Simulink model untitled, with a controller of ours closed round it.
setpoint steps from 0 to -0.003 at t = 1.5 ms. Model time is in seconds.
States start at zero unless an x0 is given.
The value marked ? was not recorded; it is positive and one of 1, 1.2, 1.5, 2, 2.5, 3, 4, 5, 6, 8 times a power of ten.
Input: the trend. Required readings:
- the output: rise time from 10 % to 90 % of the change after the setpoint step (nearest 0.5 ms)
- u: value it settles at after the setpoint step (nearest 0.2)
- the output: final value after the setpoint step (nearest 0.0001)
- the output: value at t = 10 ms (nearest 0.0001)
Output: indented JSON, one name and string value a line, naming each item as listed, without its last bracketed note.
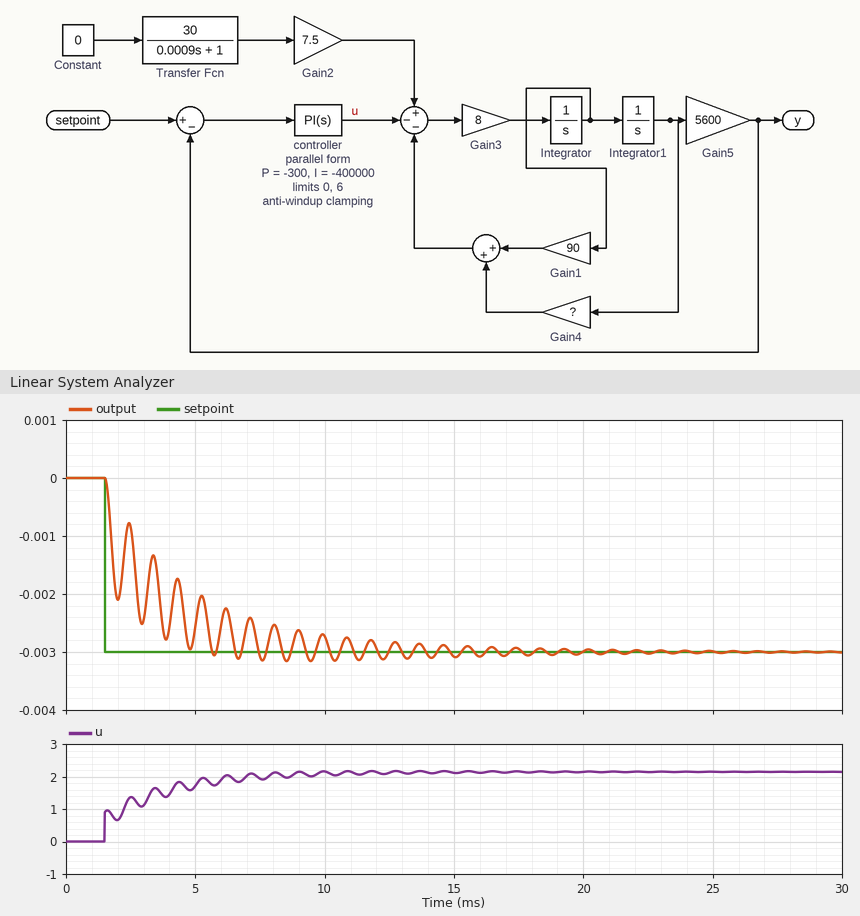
{
  "the output: rise time from 10 % to 90 % of the change after the setpoint step": "2.0 ms",
  "u: value it settles at after the setpoint step": "2.2",
  "the output: final value after the setpoint step": "-0.0030",
  "the output: value at t = 10 ms": "-0.0027"
}
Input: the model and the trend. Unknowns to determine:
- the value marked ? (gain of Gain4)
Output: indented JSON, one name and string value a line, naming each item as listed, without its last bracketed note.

{
  "the value marked ?": "4e+06"
}
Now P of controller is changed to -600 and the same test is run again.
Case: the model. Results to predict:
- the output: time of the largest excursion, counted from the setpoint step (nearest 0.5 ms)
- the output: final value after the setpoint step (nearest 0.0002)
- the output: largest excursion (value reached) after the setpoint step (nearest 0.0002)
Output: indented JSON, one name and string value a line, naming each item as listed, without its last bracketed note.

{
  "the output: time of the largest excursion, counted from the setpoint step": "5.5 ms",
  "the output: final value after the setpoint step": "-0.0030",
  "the output: largest excursion (value reached) after the setpoint step": "-0.0032"
}
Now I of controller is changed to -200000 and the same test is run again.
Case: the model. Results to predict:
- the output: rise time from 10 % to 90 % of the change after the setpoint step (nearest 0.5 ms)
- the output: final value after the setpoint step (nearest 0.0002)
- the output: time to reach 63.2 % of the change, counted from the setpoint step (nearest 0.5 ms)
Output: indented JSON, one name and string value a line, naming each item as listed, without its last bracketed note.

{
  "the output: rise time from 10 % to 90 % of the change after the setpoint step": "8.5 ms",
  "the output: final value after the setpoint step": "-0.0030",
  "the output: time to reach 63.2 % of the change, counted from the setpoint step": "1.5 ms"
}
